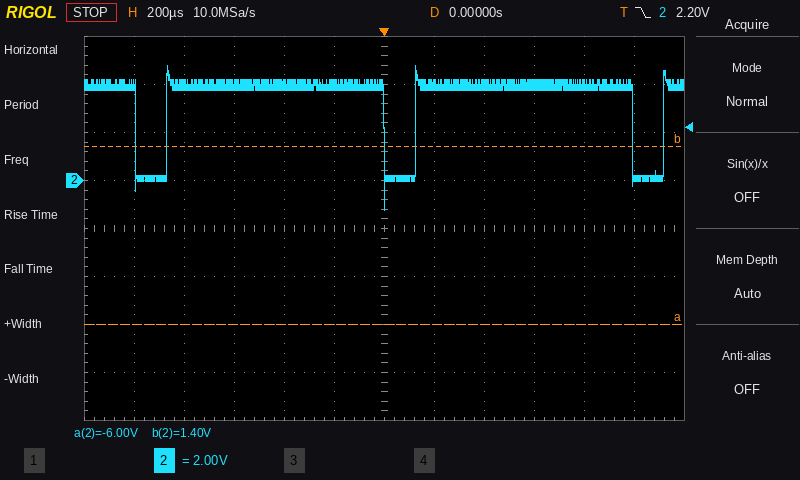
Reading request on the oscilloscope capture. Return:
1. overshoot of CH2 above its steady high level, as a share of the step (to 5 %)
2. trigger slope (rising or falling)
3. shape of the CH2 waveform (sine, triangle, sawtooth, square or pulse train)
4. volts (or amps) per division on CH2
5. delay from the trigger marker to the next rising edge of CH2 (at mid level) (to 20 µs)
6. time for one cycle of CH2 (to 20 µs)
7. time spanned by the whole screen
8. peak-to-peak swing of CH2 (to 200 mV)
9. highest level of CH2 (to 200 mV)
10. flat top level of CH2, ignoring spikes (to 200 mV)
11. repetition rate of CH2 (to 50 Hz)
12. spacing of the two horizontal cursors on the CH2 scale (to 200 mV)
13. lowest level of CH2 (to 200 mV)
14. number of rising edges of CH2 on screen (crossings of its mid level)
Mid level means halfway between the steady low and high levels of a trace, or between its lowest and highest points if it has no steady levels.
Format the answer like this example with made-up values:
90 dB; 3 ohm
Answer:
20 %; falling; pulse train; 2 V; 120 µs; 1.00 ms; 2.4 ms; 6.0 V; 4.8 V; 4.0 V; 1.00 kHz; 7.4 V; -1.2 V; 3
